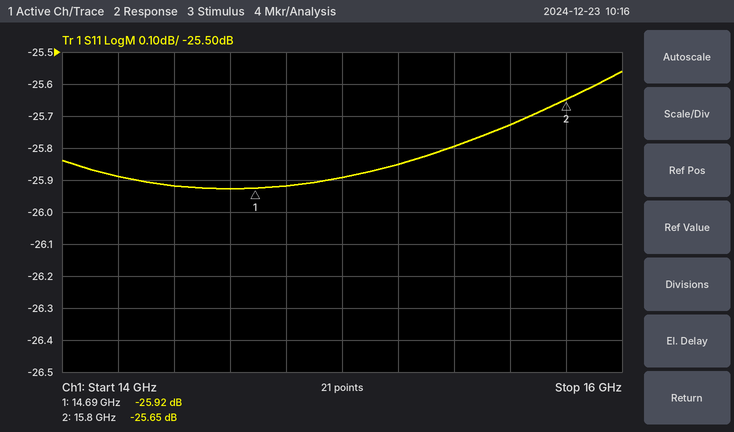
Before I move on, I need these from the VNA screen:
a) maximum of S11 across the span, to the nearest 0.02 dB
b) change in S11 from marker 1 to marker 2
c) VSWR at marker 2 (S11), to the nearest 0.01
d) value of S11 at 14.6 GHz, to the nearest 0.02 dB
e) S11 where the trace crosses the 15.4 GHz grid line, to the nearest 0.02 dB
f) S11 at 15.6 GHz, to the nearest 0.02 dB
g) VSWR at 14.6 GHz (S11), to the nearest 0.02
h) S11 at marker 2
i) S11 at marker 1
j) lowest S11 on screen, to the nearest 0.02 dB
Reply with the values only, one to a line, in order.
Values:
-25.56 dB
0.27 dB
1.11
-25.92 dB
-25.80 dB
-25.72 dB
1.10
-25.65 dB
-25.92 dB
-25.92 dB
